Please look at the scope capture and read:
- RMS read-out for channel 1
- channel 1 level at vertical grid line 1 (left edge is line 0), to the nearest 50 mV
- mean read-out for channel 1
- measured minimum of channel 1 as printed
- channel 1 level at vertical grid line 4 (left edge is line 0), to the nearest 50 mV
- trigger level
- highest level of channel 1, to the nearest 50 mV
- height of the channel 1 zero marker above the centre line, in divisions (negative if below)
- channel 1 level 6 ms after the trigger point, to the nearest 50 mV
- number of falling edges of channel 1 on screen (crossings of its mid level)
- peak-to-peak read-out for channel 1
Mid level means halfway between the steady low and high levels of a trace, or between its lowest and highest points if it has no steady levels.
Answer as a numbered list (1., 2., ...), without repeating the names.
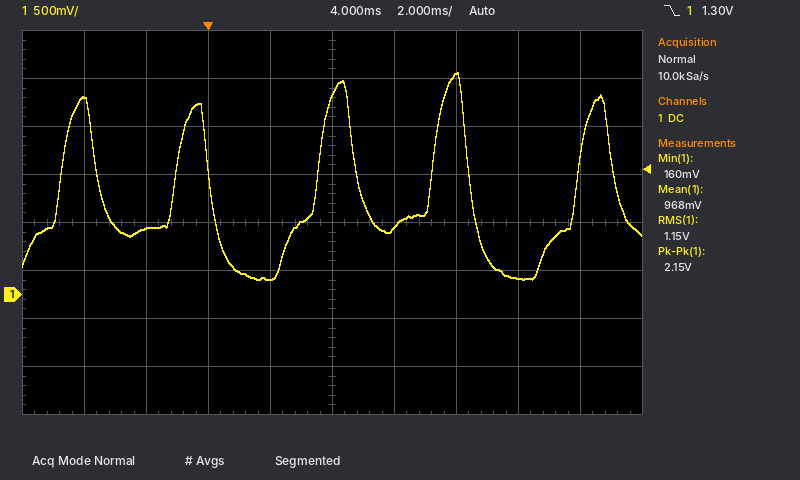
1. 1.15 V
2. 2.05 V
3. 968 mV
4. 160 mV
5. 150 mV
6. 1.30 V
7. 2.30 V
8. -1.5 div
9. 700 mV
10. 5
11. 2.15 V
